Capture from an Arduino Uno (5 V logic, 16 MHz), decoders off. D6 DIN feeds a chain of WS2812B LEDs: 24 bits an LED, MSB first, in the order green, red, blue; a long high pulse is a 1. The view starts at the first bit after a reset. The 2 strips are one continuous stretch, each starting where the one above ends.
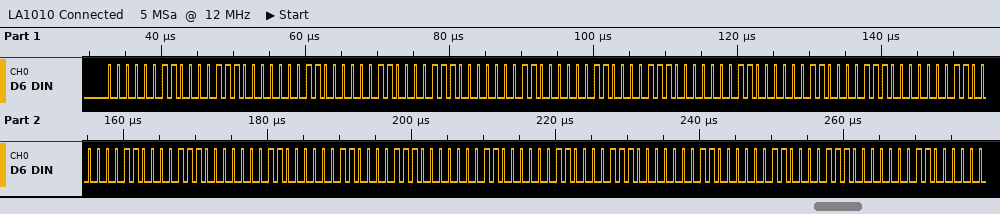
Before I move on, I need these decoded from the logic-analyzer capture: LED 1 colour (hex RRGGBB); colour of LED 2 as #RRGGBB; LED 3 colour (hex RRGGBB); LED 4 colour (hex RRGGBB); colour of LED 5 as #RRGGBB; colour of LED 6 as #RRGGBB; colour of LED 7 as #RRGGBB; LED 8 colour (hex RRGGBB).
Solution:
#0E0303
#0E0303
#0E0303
#0E0303
#0E0303
#0E0303
#0E0303
#0E0303
